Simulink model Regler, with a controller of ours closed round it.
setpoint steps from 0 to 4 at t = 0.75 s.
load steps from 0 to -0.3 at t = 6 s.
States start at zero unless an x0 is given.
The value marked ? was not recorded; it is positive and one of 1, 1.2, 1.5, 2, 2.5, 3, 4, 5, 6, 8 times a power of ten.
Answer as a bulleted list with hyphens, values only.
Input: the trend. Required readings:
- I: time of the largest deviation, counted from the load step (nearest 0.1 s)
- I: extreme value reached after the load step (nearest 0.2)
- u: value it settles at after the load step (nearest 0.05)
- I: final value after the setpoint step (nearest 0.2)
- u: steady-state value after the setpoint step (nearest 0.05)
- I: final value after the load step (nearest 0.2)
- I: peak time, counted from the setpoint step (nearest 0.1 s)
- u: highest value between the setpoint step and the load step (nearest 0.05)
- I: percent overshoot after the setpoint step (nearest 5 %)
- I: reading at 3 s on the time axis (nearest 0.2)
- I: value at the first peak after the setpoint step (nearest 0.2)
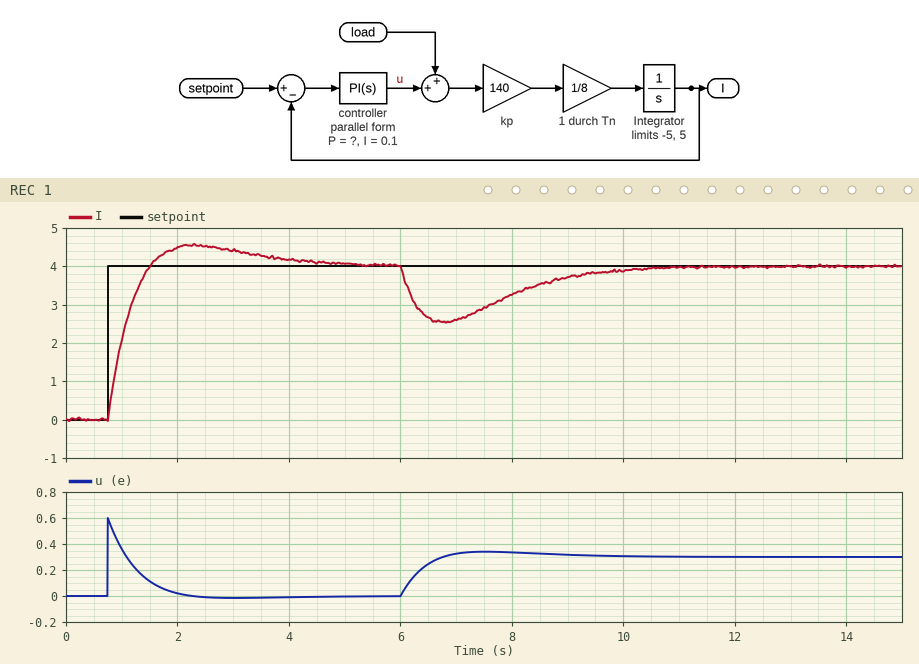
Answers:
- 0.8 s
- 2.6
- 0.30
- 4.0
- 0.00
- 4.0
- 1.5 s
- 0.60
- 15 %
- 4.4
- 4.6
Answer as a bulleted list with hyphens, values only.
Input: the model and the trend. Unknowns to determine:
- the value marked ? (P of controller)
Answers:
- 0.15
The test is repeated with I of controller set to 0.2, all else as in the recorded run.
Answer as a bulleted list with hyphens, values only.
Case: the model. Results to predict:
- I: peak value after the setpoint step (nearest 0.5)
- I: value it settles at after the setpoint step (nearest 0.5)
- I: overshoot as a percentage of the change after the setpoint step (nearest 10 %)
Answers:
- 5.0
- 4.0
- 20 %
